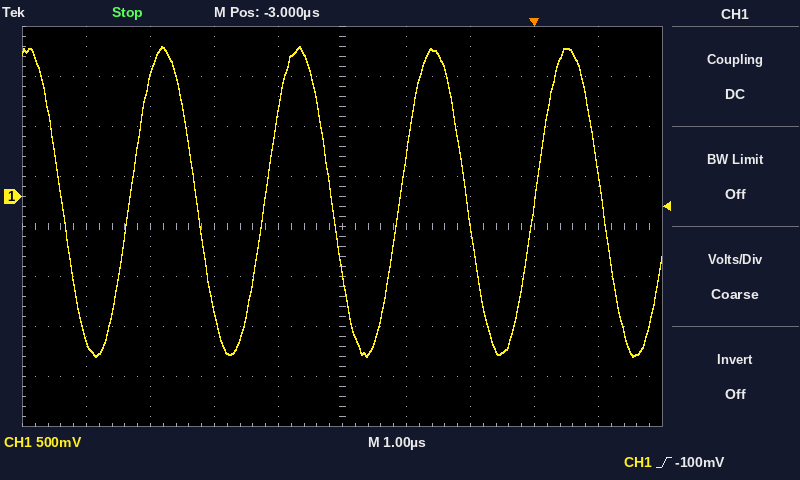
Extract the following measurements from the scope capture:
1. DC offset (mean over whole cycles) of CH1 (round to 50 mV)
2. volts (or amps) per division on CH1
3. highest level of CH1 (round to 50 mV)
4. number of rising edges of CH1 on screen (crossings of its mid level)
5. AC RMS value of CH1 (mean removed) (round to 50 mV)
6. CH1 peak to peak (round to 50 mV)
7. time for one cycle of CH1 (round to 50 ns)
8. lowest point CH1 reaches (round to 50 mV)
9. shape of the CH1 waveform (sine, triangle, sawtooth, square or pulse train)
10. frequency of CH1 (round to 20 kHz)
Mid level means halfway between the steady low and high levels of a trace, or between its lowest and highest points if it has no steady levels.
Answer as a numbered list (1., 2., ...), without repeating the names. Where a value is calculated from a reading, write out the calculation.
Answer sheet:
1. (1.50 V + (-1.60 V)) / 2 ≈ -50 mV
2. 500 mV
3. 1.50 V
4. 4
5. 3.10 V / (2√2) ≈ 1.10 V
6. 1.50 V − (-1.60 V) = 3.10 V
7. 2.10 µs
8. -1.60 V
9. sine
10. 1 / 2.10 µs ≈ 476 kHz, so 480 kHz to the nearest 20 kHz
